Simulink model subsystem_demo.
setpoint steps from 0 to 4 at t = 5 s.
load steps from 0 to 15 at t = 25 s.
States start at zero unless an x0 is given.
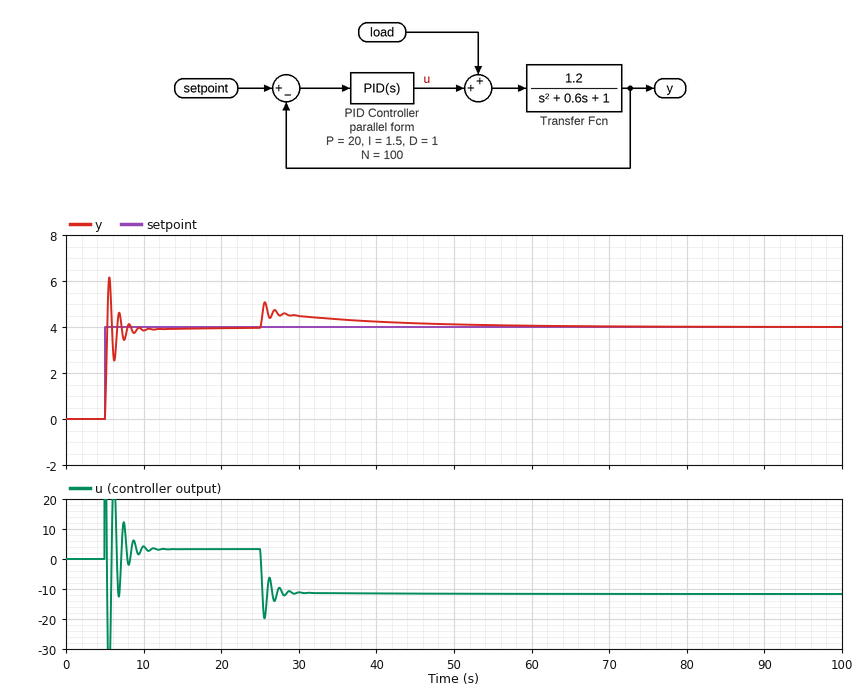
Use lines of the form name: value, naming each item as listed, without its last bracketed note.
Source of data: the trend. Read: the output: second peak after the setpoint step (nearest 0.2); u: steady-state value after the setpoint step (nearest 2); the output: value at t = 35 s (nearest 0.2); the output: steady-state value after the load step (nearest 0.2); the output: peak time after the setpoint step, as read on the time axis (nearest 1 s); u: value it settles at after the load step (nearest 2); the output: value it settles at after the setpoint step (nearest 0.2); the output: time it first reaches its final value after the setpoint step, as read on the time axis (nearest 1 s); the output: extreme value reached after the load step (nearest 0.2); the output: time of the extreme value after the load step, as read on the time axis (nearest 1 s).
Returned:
the output: second peak after the setpoint step: 4.6
u: steady-state value after the setpoint step: 4
the output: value at t = 35 s: 4.4
the output: steady-state value after the load step: 4.0
the output: peak time after the setpoint step, as read on the time axis: 6 s
u: value it settles at after the load step: -12
the output: value it settles at after the setpoint step: 4.0
the output: time it first reaches its final value after the setpoint step, as read on the time axis: 5 s
the output: extreme value reached after the load step: 5.0
the output: time of the extreme value after the load step, as read on the time axis: 26 s
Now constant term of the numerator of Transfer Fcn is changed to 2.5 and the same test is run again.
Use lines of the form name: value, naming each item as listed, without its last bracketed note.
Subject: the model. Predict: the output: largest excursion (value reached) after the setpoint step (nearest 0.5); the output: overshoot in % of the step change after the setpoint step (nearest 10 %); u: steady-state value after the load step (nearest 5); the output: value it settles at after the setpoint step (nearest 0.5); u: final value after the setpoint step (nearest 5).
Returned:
the output: largest excursion (value reached) after the setpoint step: 6.0
the output: overshoot in % of the step change after the setpoint step: 50 %
u: steady-state value after the load step: -15
the output: value it settles at after the setpoint step: 4.0
u: final value after the setpoint step: 0
